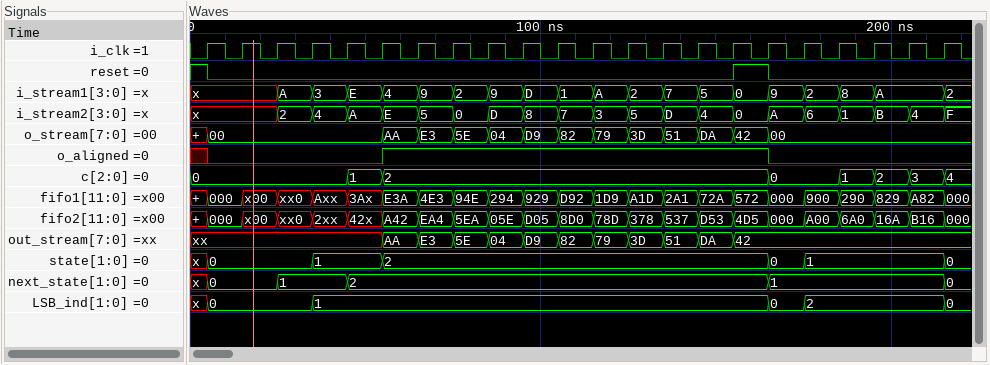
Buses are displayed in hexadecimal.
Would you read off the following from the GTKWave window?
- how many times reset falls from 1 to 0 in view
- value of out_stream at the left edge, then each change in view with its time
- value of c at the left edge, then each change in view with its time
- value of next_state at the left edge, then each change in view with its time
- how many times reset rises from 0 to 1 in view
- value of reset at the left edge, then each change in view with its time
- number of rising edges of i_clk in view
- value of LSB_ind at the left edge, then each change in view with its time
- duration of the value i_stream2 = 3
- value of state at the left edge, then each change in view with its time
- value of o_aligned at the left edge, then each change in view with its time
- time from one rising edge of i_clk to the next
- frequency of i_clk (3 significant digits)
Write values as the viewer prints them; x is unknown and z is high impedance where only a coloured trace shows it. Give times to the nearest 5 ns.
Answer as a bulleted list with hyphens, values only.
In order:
- 2
- xx, AA at 55 ns, E3 at 65 ns, 5E at 75 ns, 04 at 85 ns, D9 at 95 ns, 82 at 105 ns, 79 at 115 ns, 3D at 125 ns, 51 at 135 ns, DA at 145 ns, 42 at 155 ns
- 0, 1 at 45 ns, 2 at 55 ns, 0 at 165 ns, 1 at 185 ns, 2 at 195 ns, 3 at 205 ns, 4 at 215 ns
- x, 0 at 5 ns, 1 at 25 ns, 2 at 45 ns, 1 at 165 ns, 0 at 215 ns
- 1
- 1, 0 at 5 ns, 1 at 155 ns, 0 at 165 ns
- 22
- x, 0 at 5 ns, 1 at 35 ns, 0 at 165 ns, 2 at 175 ns, 0 at 215 ns
- 10 ns
- x, 0 at 5 ns, 1 at 35 ns, 2 at 55 ns, 0 at 165 ns, 1 at 175 ns, 0 at 215 ns
- x, 0 at 5 ns, 1 at 55 ns, 0 at 165 ns
- 10 ns
- 100 MHz
